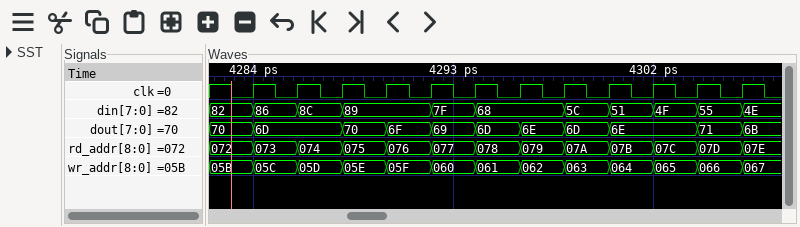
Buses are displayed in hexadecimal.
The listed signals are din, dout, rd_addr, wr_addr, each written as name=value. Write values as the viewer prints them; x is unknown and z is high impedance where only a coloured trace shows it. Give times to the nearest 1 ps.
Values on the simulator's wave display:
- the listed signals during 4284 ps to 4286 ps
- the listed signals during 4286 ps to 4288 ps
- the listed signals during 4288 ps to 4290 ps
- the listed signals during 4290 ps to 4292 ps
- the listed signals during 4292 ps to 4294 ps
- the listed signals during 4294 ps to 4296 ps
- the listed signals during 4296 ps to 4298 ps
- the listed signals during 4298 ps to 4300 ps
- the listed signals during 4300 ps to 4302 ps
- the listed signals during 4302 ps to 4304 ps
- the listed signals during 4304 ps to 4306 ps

din=86, dout=6D, rd_addr=073, wr_addr=05C
din=8C, dout=6D, rd_addr=074, wr_addr=05D
din=89, dout=70, rd_addr=075, wr_addr=05E
din=89, dout=6F, rd_addr=076, wr_addr=05F
din=7F, dout=69, rd_addr=077, wr_addr=060
din=68, dout=6D, rd_addr=078, wr_addr=061
din=68, dout=6E, rd_addr=079, wr_addr=062
din=5C, dout=6D, rd_addr=07A, wr_addr=063
din=51, dout=6E, rd_addr=07B, wr_addr=064
din=4F, dout=6E, rd_addr=07C, wr_addr=065
din=55, dout=71, rd_addr=07D, wr_addr=066
